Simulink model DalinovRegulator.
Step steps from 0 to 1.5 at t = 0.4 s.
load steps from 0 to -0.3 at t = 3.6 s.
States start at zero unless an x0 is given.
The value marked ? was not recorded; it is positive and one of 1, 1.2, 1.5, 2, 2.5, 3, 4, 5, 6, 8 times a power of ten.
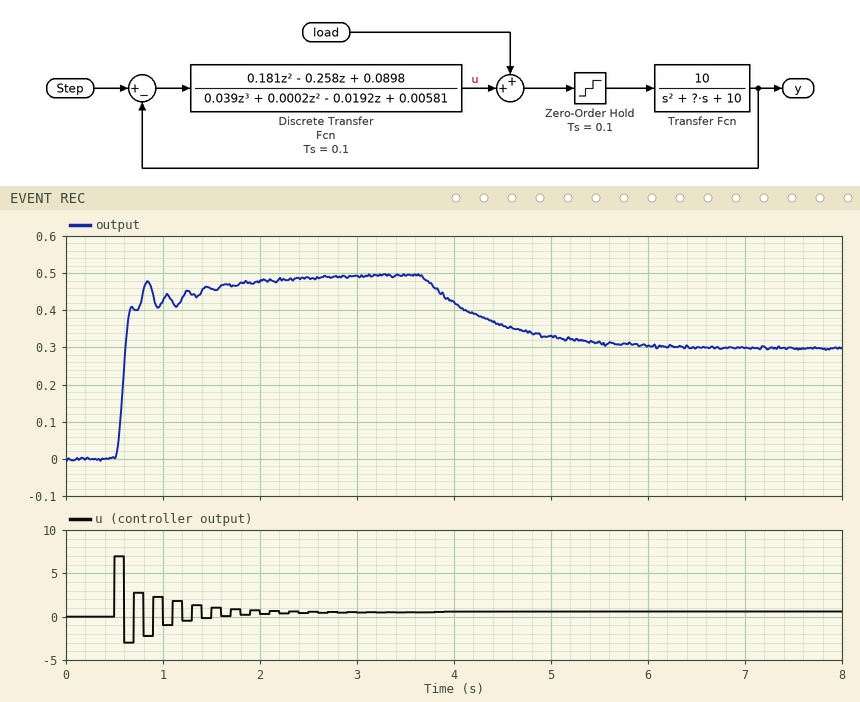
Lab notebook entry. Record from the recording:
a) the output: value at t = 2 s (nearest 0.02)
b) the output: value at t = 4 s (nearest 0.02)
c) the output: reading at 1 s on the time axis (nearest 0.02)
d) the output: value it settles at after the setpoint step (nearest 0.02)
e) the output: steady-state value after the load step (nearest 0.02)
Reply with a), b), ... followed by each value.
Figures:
a) 0.48
b) 0.42
c) 0.42
d) 0.50
e) 0.30
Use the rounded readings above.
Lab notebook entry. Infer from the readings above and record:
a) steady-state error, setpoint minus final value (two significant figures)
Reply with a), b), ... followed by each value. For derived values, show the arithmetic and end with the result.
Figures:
a) 1.5 - 0.5 = 1.0
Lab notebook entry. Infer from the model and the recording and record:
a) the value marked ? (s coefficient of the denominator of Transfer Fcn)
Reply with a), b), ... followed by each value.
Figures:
a) 10
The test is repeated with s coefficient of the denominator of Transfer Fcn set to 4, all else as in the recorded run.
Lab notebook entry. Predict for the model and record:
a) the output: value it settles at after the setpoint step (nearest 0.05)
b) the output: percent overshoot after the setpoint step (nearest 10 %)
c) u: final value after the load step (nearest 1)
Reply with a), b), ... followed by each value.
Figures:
a) 0.50
b) 70 %
c) 1
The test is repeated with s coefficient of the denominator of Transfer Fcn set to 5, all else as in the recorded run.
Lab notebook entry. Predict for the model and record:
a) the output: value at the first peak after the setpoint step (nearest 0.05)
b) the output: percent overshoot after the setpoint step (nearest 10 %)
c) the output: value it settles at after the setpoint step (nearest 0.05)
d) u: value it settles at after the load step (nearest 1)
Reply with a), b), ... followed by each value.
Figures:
a) 0.75
b) 50 %
c) 0.50
d) 1
